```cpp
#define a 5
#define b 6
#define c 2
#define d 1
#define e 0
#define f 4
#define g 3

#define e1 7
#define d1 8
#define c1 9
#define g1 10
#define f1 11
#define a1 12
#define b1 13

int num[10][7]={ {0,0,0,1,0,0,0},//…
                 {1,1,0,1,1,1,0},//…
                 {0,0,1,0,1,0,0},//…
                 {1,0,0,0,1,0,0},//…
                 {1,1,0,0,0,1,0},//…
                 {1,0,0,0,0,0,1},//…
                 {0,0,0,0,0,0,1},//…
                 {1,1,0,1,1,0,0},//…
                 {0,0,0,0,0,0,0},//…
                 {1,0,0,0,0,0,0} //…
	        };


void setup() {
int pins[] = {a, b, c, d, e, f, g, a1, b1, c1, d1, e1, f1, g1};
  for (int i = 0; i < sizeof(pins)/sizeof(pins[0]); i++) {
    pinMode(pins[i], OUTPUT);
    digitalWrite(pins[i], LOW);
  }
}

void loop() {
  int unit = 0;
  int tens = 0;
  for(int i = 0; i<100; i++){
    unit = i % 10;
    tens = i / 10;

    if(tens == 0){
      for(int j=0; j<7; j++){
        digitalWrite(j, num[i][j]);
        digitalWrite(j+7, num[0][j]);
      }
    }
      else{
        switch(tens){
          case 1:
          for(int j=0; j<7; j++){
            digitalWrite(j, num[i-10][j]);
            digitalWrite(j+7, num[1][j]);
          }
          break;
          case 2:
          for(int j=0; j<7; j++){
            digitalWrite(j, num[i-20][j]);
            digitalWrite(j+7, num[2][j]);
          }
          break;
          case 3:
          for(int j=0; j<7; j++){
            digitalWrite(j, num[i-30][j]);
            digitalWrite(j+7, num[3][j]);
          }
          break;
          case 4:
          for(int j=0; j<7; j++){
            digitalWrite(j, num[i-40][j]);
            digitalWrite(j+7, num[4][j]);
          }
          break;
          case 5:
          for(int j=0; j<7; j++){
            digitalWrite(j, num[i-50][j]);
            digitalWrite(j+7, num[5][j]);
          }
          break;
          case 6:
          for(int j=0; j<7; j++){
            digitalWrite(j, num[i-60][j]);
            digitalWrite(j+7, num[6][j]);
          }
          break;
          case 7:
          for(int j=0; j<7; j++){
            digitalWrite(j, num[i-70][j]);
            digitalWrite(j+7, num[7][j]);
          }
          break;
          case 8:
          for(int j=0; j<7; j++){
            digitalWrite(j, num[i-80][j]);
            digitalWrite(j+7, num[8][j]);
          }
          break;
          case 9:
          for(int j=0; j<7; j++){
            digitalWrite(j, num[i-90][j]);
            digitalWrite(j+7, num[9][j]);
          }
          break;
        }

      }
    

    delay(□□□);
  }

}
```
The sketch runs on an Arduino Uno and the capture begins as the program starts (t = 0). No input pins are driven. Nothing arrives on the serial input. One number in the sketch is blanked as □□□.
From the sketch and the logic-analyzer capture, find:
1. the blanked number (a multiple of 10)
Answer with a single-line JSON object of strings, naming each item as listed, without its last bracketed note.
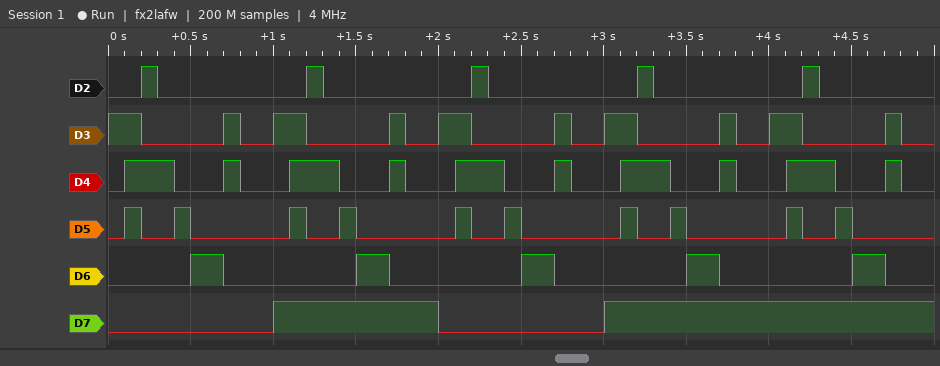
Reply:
{"the blanked number": "100"}
